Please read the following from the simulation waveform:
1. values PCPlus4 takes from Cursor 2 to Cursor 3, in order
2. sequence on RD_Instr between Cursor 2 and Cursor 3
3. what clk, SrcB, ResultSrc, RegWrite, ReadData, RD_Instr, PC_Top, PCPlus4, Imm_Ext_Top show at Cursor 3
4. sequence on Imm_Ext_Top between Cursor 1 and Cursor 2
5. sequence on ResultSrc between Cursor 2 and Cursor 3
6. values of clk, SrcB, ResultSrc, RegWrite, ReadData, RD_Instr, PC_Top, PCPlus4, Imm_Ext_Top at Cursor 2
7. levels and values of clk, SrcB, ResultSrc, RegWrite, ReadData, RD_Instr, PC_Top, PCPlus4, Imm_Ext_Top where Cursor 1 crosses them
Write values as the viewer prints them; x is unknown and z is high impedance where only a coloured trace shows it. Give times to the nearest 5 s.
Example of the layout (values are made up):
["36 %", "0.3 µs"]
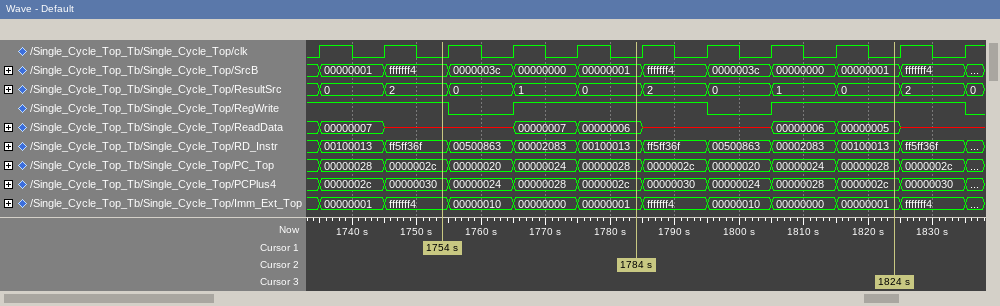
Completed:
["0000002c, 00000030, 00000024, 00000028, 0000002c", "00100013, ff5ff36f, 00500863, 00002083, 00100013", "clk=0, SrcB=00000001, ResultSrc=0, RegWrite=1, ReadData=00000005, RD_Instr=00100013, PC_Top=00000028, PCPlus4=0000002c, Imm_Ext_Top=00000001", "fffffff4, 00000010, 00000000, 00000001", "0, 2, 0, 1, 0", "clk=0, SrcB=00000001, ResultSrc=0, RegWrite=1, ReadData=00000006, RD_Instr=00100013, PC_Top=00000028, PCPlus4=0000002c, Imm_Ext_Top=00000001", "clk=0, SrcB=fffffff4, ResultSrc=2, RegWrite=1, ReadData=x, RD_Instr=ff5ff36f, PC_Top=0000002c, PCPlus4=00000030, Imm_Ext_Top=fffffff4"]
